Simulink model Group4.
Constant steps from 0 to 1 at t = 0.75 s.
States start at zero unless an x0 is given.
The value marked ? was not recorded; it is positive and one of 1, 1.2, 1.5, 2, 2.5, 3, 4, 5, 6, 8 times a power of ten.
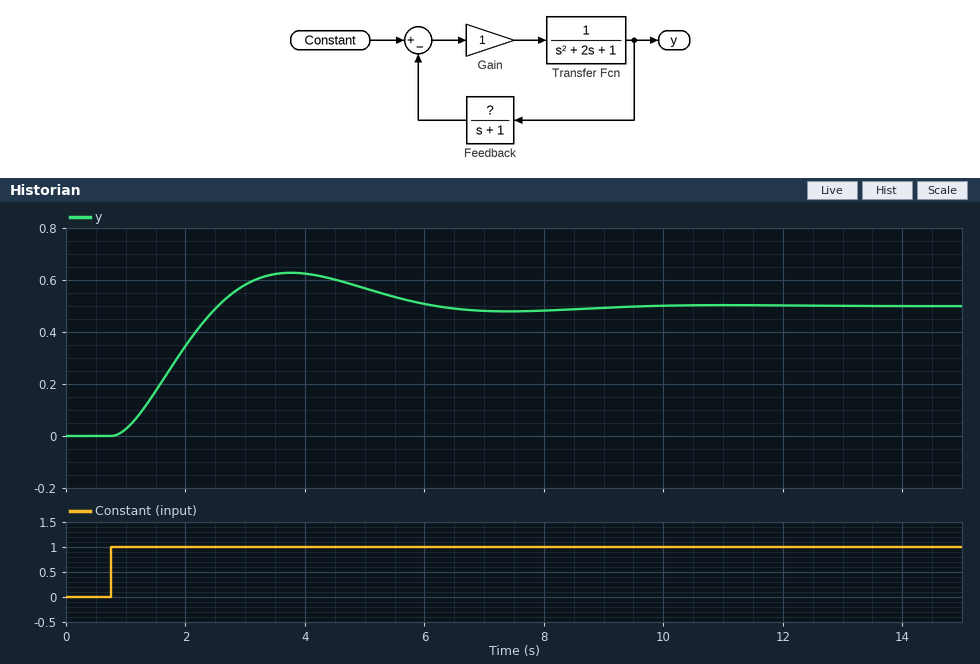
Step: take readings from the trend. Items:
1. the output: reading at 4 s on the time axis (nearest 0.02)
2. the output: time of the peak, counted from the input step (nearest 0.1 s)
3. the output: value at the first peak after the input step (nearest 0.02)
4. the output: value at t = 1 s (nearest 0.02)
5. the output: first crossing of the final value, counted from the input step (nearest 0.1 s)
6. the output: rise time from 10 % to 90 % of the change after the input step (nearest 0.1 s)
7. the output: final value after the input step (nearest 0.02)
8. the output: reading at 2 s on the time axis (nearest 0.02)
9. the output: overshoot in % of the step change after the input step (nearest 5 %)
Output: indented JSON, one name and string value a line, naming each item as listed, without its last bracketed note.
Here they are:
{
  "the output: reading at 4 s on the time axis": "0.62",
  "the output: time of the peak, counted from the input step": "3.0 s",
  "the output: value at the first peak after the input step": "0.62",
  "the output: value at t = 1 s": "0.02",
  "the output: first crossing of the final value, counted from the input step": "1.8 s",
  "the output: rise time from 10 % to 90 % of the change after the input step": "1.2 s",
  "the output: final value after the input step": "0.50",
  "the output: reading at 2 s on the time axis": "0.34",
  "the output: overshoot in % of the step change after the input step": "25 %"
}
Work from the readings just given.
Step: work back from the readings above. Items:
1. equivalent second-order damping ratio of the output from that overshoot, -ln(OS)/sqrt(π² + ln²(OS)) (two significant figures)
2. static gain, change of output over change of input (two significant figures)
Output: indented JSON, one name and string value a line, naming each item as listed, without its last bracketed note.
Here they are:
{
  "equivalent second-order damping ratio of the output from that overshoot, -ln(OS)/sqrt(π² + ln²(OS))": "0.40",
  "static gain, change of output over change of input": "0.50"
}
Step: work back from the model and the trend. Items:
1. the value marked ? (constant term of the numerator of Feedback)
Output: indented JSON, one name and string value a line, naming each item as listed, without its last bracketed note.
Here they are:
{
  "the value marked ?": "1"
}
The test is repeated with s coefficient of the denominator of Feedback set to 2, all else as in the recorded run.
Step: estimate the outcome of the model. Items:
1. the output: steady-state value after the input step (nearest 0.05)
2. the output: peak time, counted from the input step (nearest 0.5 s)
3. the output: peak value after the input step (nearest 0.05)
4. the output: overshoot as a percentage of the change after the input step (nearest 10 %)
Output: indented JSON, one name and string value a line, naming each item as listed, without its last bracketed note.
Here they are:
{
  "the output: steady-state value after the input step": "0.50",
  "the output: peak time, counted from the input step": "3.5 s",
  "the output: peak value after the input step": "0.70",
  "the output: overshoot as a percentage of the change after the input step": "40 %"
}
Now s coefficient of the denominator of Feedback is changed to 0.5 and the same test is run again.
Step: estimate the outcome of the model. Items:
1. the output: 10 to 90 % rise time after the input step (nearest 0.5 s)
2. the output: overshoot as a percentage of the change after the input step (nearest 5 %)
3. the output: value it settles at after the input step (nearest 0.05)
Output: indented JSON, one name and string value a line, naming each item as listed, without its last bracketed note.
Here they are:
{
  "the output: 10 to 90 % rise time after the input step": "1.5 s",
  "the output: overshoot as a percentage of the change after the input step": "15 %",
  "the output: value it settles at after the input step": "0.50"
}
